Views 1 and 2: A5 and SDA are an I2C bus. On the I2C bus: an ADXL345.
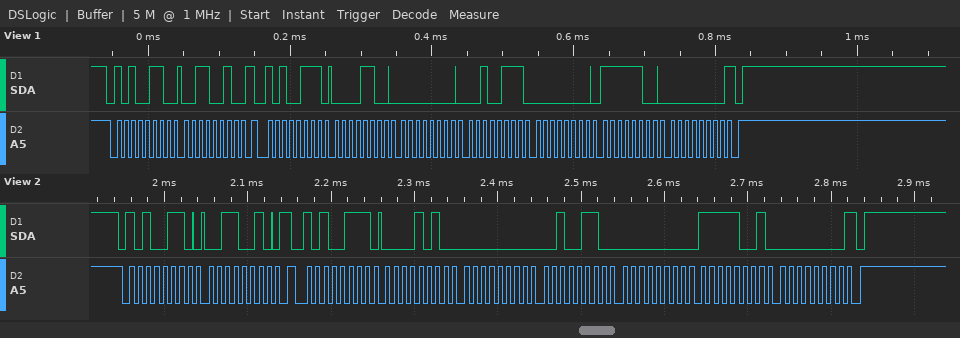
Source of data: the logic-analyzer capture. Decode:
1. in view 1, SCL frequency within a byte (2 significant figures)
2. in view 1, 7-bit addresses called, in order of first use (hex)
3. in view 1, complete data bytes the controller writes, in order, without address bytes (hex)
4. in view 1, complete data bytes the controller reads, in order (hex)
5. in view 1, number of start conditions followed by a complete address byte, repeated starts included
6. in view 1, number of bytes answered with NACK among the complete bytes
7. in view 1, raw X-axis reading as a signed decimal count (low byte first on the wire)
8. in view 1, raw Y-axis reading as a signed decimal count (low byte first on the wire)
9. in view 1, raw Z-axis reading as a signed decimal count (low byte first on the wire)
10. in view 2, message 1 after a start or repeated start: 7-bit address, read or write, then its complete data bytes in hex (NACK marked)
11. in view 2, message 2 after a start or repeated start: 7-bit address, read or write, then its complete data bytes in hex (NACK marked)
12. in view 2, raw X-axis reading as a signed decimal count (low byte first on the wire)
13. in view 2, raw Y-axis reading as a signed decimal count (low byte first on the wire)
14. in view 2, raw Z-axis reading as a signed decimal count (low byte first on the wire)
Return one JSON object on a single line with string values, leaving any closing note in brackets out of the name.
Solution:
{"in view 1, SCL frequency within a byte": "100 kHz", "in view 1, 7-bit addresses called, in order of first use": "0x53", "in view 1, complete data bytes the controller writes, in order, without address bytes": "32", "in view 1, complete data bytes the controller reads, in order": "0C 00 27 00 FC 00", "in view 1, number of start conditions followed by a complete address byte, repeated starts included": "2", "in view 1, number of bytes answered with NACK among the complete bytes": "1", "in view 1, raw X-axis reading as a signed decimal count": "12", "in view 1, raw Y-axis reading as a signed decimal count": "39", "in view 1, raw Z-axis reading as a signed decimal count": "252", "in view 2, message 1 after a start or repeated start: 7-bit address, read or write, then its complete data bytes in hex": "0x53 write: 32", "in view 2, message 2 after a start or repeated start: 7-bit address, read or write, then its complete data bytes in hex": "0x53 read: 0A 00 26 00 F9 00 NACK", "in view 2, raw X-axis reading as a signed decimal count": "10", "in view 2, raw Y-axis reading as a signed decimal count": "38", "in view 2, raw Z-axis reading as a signed decimal count": "249"}
